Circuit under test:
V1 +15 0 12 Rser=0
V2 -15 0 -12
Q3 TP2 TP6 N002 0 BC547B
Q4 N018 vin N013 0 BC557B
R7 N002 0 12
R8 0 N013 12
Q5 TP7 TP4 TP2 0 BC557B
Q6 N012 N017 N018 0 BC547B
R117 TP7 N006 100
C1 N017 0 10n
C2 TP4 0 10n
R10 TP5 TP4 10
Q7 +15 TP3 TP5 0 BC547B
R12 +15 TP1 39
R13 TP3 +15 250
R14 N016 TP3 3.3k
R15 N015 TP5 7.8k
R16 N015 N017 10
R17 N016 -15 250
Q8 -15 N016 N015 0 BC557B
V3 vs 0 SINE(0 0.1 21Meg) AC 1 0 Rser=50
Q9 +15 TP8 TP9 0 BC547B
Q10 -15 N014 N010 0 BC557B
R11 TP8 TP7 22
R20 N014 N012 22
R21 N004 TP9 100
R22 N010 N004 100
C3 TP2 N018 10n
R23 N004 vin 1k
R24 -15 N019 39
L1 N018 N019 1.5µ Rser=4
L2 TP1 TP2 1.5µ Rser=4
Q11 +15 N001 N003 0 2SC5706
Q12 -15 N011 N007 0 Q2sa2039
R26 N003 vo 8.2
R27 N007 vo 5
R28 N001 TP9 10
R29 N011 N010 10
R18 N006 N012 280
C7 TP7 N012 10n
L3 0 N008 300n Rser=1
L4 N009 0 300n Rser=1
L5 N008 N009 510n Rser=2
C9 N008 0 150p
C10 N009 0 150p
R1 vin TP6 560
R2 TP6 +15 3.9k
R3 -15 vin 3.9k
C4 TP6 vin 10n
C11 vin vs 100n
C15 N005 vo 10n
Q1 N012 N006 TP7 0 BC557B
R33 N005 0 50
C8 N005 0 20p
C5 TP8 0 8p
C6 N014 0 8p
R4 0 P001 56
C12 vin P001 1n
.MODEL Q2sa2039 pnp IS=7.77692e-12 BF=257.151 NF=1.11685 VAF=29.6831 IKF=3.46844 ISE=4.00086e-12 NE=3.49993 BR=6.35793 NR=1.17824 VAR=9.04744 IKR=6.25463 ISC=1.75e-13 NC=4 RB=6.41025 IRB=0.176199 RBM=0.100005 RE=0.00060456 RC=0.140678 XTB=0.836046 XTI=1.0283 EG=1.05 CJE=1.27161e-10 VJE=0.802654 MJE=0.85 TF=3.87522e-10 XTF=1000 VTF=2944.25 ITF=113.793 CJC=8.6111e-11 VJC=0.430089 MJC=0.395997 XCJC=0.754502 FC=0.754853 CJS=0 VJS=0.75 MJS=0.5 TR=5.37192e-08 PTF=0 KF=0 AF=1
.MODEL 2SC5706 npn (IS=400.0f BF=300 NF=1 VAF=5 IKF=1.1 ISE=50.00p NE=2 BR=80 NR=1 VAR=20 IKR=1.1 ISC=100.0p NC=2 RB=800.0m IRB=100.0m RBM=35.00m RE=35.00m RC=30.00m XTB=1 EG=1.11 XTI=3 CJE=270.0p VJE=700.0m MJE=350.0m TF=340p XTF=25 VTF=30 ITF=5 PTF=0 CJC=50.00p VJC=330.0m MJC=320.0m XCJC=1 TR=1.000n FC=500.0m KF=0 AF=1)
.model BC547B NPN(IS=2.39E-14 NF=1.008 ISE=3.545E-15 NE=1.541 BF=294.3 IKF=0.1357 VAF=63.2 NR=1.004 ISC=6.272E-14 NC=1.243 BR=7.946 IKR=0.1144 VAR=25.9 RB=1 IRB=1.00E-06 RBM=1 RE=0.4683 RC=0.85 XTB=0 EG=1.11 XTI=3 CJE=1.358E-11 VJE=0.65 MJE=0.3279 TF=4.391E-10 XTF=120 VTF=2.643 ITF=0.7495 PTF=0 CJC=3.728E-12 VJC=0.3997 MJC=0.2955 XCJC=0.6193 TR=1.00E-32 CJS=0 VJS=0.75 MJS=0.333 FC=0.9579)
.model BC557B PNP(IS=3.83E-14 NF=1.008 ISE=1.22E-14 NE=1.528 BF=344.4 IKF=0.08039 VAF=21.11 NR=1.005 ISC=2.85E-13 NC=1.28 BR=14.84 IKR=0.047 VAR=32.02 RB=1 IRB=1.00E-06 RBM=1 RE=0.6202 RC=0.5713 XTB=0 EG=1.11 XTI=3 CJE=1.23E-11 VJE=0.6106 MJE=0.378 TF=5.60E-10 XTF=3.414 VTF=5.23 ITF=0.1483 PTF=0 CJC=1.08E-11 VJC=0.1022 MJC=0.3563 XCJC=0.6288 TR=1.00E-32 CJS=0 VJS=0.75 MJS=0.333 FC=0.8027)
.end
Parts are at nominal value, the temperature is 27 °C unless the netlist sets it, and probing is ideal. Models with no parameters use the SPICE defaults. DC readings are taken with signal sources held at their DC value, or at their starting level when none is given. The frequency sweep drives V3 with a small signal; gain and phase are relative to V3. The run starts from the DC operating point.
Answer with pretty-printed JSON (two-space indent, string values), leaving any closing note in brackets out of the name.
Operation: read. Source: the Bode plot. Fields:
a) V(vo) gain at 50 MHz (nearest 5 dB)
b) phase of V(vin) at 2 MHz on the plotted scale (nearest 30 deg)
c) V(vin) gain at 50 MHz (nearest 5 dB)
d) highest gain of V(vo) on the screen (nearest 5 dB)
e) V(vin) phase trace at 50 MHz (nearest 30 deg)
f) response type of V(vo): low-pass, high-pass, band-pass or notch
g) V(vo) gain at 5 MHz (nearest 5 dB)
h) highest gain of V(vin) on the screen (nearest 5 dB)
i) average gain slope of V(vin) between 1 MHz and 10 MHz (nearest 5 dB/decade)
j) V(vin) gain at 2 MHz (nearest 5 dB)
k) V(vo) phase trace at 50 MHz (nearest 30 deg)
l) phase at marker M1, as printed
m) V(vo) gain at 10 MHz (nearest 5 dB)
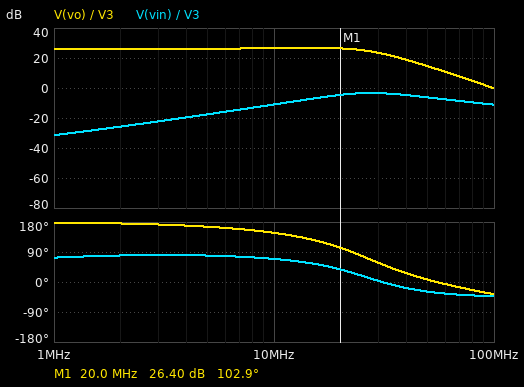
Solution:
{
  "V(vo) gain at 50 MHz": "15 dB",
  "phase of V(vin) at 2 MHz on the plotted scale": "90 deg",
  "V(vin) gain at 50 MHz": "-5 dB",
  "highest gain of V(vo) on the screen": "25 dB",
  "V(vin) phase trace at 50 MHz": "-30 deg",
  "response type of V(vo): low-pass, high-pass, band-pass or notch": "low-pass",
  "V(vo) gain at 5 MHz": "25 dB",
  "highest gain of V(vin) on the screen": "-5 dB",
  "average gain slope of V(vin) between 1 MHz and 10 MHz": "20 dB/decade",
  "V(vin) gain at 2 MHz": "-25 dB",
  "V(vo) phase trace at 50 MHz": "0 deg",
  "phase at marker M1, as printed": "102.9 deg",
  "V(vo) gain at 10 MHz": "25 dB"
}
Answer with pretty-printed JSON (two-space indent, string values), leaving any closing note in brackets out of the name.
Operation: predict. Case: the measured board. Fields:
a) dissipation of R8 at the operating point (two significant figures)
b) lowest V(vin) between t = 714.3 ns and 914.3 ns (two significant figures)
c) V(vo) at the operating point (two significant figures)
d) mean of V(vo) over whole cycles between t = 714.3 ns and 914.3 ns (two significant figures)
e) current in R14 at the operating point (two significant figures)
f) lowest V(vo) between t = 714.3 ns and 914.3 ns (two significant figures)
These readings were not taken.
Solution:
{
  "dissipation of R8 at the operating point": "880 µW",
  "lowest V(vin) between t = 714.3 ns and 914.3 ns": "-850 mV",
  "V(vo) at the operating point": "-780 mV",
  "mean of V(vo) over whole cycles between t = 714.3 ns and 914.3 ns": "-780 mV",
  "current in R14 at the operating point": "6.3 mA",
  "lowest V(vo) between t = 714.3 ns and 914.3 ns": "-2.8 V"
}
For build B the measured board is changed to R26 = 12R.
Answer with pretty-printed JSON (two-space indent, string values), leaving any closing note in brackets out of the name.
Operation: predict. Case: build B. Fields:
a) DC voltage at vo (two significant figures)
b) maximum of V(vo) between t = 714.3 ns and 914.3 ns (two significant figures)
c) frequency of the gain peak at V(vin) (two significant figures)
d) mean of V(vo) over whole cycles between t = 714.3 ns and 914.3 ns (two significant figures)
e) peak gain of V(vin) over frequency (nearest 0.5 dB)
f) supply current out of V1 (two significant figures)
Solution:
{
  "DC voltage at vo": "-800 mV",
  "maximum of V(vo) between t = 714.3 ns and 914.3 ns": "1.1 V",
  "frequency of the gain peak at V(vin)": "27 MHz",
  "mean of V(vo) over whole cycles between t = 714.3 ns and 914.3 ns": "-820 mV",
  "peak gain of V(vin) over frequency": "-3.5 dB",
  "supply current out of V1": "65 mA"
}
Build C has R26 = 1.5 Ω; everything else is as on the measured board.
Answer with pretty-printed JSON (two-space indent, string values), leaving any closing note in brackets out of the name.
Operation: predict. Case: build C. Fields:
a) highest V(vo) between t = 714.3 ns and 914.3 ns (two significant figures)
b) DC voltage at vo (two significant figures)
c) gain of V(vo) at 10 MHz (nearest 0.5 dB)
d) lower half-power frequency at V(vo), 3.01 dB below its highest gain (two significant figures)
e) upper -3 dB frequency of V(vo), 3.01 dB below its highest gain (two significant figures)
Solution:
{
  "highest V(vo) between t = 714.3 ns and 914.3 ns": "1.5 V",
  "DC voltage at vo": "-720 mV",
  "gain of V(vo) at 10 MHz": "27.0 dB",
  "lower half-power frequency at V(vo), 3.01 dB below its highest gain": "37 kHz",
  "upper -3 dB frequency of V(vo), 3.01 dB below its highest gain": "30 MHz"
}
